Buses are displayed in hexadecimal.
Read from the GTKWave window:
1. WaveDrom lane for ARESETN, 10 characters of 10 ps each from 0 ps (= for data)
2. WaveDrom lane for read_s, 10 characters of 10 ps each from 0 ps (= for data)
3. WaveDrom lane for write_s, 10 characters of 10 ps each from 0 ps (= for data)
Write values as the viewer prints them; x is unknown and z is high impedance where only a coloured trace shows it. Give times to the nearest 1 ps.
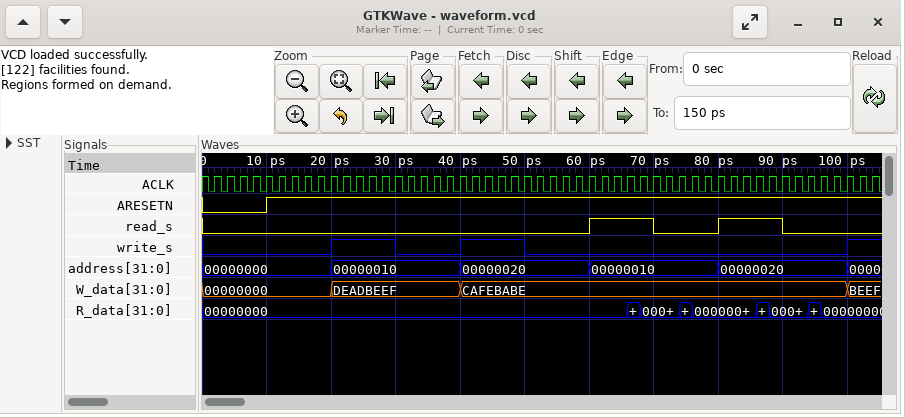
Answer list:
{name: 'ARESETN', wave: '01........'}
{name: 'read_s', wave: '0.....1010'}
{name: 'write_s', wave: '0.1010....'}
